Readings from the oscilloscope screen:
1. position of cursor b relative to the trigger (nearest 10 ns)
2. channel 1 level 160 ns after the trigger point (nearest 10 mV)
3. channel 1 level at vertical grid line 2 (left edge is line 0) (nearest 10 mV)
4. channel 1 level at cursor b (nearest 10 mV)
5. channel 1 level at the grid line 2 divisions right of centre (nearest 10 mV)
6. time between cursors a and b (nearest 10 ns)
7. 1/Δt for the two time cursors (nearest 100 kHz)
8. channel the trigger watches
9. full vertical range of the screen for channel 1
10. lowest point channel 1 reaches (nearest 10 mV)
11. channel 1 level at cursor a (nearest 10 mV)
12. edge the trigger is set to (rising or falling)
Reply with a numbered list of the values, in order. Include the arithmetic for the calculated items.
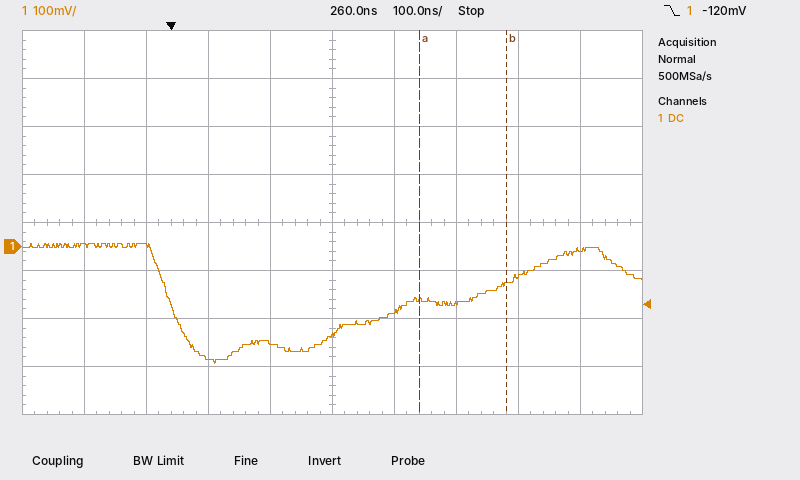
1. +540 ns
2. -200 mV
3. 0 mV
4. -80 mV
5. -120 mV
6. 140 ns
7. 1 / 140 ns ≈ 7.1 MHz
8. channel 1
9. 800 mV
10. -240 mV
11. -110 mV
12. falling
